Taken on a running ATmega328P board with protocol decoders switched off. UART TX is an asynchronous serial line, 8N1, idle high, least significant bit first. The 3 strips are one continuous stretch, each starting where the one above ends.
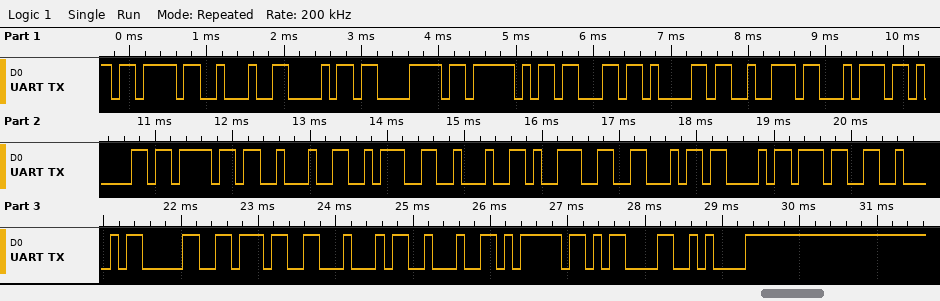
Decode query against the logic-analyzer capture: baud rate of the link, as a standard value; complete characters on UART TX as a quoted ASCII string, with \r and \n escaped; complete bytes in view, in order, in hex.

9600 baud
"{\"hx_cartao\":\"9FC7B07D\"}\r\n"
7B 22 68 78 5F 63 61 72 74 61 6F 22 3A 22 39 46 43 37 42 30 37 44 22 7D 0D 0A
